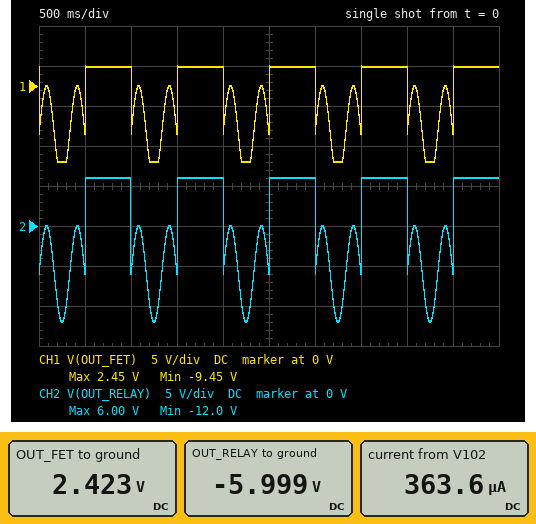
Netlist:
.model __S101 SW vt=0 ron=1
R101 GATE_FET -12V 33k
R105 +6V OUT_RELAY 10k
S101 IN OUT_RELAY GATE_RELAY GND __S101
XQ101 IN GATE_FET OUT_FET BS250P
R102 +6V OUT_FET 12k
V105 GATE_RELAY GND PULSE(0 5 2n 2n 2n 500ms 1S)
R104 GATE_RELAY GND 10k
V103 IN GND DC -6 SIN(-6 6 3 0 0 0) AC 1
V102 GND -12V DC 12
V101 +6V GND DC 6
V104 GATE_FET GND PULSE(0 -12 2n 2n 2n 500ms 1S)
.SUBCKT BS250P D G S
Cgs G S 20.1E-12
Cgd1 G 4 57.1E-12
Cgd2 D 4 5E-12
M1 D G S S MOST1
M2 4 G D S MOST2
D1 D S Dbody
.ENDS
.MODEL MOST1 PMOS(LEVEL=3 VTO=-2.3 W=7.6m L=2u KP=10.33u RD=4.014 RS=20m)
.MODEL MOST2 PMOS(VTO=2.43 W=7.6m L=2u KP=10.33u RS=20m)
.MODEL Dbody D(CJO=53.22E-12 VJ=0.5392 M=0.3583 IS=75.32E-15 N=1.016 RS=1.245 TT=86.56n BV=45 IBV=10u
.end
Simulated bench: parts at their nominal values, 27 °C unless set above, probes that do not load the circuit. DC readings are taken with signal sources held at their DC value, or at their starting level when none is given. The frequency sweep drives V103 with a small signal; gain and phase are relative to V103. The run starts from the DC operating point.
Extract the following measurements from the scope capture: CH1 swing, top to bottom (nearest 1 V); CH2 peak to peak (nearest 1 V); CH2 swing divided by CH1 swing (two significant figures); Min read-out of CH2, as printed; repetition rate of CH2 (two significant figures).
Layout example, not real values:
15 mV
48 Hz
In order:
12 V
18 V
1.5
-12.0 V
1.0 Hz
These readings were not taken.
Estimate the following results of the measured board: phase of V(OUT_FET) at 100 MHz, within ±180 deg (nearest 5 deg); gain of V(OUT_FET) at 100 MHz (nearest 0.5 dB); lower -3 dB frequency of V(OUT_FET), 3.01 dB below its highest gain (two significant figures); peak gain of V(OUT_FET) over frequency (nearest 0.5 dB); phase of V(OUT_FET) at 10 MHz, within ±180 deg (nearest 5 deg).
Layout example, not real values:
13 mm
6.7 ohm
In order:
10 deg
-7.0 dB
18 MHz
-7.0 dB
60 deg
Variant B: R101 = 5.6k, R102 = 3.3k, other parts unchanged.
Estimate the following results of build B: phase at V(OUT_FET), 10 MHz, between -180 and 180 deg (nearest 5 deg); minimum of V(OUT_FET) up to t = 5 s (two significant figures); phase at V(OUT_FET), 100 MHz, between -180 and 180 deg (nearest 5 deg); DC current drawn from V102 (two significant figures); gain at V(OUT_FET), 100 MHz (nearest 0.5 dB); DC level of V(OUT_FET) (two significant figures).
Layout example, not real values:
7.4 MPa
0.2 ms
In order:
75 deg
-9.2 V
20 deg
2.1 mA
-7.5 dB
2.5 V
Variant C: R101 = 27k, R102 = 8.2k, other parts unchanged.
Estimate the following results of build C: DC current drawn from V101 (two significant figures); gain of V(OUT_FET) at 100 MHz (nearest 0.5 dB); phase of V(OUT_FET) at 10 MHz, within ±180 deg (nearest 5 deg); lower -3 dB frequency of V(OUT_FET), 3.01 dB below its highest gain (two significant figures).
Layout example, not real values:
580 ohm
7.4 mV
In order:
1.6 mA
-7.0 dB
65 deg
22 MHz
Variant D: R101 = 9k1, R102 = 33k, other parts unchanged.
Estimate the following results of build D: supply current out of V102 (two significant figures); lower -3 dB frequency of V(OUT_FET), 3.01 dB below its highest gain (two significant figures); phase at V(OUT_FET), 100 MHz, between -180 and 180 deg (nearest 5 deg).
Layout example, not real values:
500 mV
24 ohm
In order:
1.3 mA
11 MHz
5 deg
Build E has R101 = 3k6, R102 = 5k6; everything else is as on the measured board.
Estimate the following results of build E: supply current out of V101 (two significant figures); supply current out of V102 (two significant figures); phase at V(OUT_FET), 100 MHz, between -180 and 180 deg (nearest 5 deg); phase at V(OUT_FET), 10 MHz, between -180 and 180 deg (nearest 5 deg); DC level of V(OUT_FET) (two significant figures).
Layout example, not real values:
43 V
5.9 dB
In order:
1.8 mA
3.3 mA
15 deg
70 deg
2.5 V
